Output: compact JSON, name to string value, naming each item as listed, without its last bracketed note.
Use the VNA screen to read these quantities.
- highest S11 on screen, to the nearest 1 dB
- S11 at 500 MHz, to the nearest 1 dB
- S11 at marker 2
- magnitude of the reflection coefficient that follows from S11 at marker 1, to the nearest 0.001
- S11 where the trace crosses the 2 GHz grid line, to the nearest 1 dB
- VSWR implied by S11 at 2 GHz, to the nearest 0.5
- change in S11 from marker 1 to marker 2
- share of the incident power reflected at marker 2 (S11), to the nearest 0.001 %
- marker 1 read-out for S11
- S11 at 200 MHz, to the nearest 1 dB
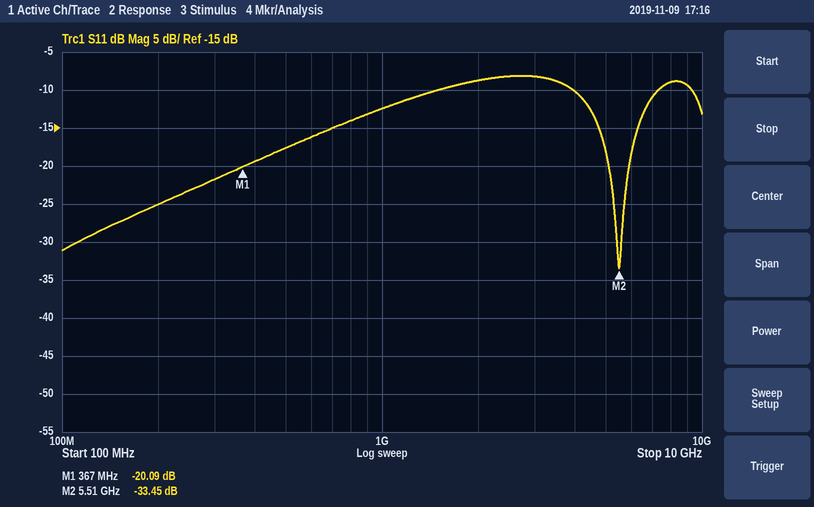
{"highest S11 on screen, to the nearest 1 dB": "-8 dB", "S11 at 500 MHz, to the nearest 1 dB": "-18 dB", "S11 at marker 2": "-33.45 dB", "magnitude of the reflection coefficient that follows from S11 at marker 1, to the nearest 0.001": "0.099", "S11 where the trace crosses the 2 GHz grid line, to the nearest 1 dB": "-9 dB", "VSWR implied by S11 at 2 GHz, to the nearest 0.5": "2.0", "change in S11 from marker 1 to marker 2": "-13.36 dB", "share of the incident power reflected at marker 2 (S11), to the nearest 0.001 %": "0.045 %", "marker 1 read-out for S11": "-20.09 dB", "S11 at 200 MHz, to the nearest 1 dB": "-25 dB"}
